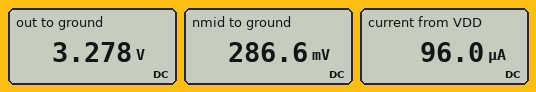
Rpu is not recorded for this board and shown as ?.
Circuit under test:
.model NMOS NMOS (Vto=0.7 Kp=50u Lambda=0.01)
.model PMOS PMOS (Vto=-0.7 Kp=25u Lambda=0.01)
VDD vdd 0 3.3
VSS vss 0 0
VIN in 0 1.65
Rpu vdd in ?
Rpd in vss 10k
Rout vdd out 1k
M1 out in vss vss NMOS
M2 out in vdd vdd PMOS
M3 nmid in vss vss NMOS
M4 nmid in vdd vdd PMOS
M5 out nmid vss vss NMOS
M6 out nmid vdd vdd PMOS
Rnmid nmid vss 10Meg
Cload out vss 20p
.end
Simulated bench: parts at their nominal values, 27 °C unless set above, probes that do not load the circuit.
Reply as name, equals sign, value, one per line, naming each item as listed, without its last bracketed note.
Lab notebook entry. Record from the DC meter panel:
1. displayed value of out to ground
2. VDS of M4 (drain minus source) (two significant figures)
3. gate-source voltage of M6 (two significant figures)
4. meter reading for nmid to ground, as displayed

displayed value of out to ground = 3.278 V
VDS of M4 (drain minus source) = -3.0 V
gate-source voltage of M6 = -3.0 V
meter reading for nmid to ground, as displayed = 286.6 mV
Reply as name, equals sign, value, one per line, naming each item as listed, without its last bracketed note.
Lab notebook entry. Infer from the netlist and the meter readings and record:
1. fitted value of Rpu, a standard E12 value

fitted value of Rpu, a standard E12 value = 27 kΩ
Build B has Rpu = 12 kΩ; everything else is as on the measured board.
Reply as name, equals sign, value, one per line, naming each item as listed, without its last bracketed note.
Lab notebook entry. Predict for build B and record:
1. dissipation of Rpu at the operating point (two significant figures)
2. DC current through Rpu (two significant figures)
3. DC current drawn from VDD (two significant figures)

dissipation of Rpu at the operating point = 230 µW
DC current through Rpu = 140 µA
DC current drawn from VDD = 170 µA
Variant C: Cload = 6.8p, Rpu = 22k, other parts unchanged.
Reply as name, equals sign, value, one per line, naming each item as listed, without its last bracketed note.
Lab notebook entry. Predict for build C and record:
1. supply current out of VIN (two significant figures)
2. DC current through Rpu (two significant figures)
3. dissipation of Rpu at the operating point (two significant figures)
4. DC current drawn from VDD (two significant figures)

supply current out of VIN = 90 µA
DC current through Rpu = 75 µA
dissipation of Rpu at the operating point = 120 µW
DC current drawn from VDD = 110 µA
